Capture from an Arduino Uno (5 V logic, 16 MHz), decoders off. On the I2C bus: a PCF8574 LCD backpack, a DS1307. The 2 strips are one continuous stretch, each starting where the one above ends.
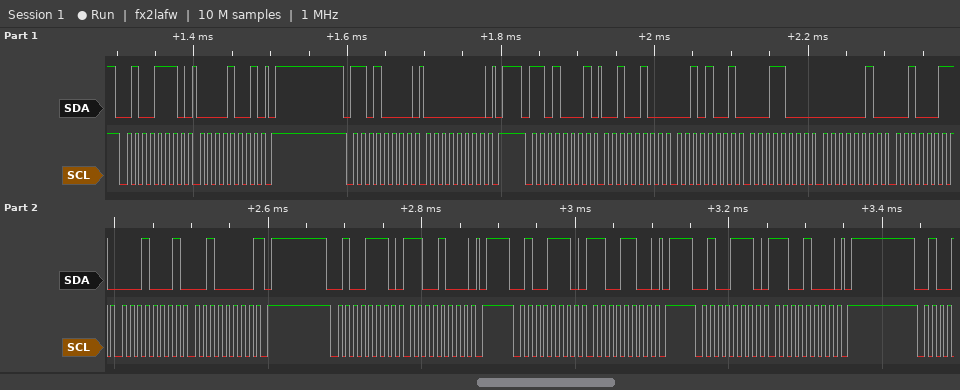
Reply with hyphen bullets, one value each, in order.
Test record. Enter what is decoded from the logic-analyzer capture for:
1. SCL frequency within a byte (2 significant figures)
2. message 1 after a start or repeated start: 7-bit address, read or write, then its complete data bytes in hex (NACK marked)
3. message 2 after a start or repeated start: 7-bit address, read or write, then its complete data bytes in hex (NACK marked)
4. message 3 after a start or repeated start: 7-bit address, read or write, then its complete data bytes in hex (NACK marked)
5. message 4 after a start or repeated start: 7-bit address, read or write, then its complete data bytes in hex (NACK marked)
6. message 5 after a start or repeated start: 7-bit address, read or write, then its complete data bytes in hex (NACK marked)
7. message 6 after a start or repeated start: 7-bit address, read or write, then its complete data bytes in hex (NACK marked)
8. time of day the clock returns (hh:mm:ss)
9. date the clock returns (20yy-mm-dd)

- 100 kHz
- 0x27 write: 09
- 0x68 write: 00
- 0x68 read: 24 29 18 02 23 11 20 NACK
- 0x27 write: C8
- 0x27 write: CC
- 0x27 write: C8
- 18:29:24
- 2020-11-23
